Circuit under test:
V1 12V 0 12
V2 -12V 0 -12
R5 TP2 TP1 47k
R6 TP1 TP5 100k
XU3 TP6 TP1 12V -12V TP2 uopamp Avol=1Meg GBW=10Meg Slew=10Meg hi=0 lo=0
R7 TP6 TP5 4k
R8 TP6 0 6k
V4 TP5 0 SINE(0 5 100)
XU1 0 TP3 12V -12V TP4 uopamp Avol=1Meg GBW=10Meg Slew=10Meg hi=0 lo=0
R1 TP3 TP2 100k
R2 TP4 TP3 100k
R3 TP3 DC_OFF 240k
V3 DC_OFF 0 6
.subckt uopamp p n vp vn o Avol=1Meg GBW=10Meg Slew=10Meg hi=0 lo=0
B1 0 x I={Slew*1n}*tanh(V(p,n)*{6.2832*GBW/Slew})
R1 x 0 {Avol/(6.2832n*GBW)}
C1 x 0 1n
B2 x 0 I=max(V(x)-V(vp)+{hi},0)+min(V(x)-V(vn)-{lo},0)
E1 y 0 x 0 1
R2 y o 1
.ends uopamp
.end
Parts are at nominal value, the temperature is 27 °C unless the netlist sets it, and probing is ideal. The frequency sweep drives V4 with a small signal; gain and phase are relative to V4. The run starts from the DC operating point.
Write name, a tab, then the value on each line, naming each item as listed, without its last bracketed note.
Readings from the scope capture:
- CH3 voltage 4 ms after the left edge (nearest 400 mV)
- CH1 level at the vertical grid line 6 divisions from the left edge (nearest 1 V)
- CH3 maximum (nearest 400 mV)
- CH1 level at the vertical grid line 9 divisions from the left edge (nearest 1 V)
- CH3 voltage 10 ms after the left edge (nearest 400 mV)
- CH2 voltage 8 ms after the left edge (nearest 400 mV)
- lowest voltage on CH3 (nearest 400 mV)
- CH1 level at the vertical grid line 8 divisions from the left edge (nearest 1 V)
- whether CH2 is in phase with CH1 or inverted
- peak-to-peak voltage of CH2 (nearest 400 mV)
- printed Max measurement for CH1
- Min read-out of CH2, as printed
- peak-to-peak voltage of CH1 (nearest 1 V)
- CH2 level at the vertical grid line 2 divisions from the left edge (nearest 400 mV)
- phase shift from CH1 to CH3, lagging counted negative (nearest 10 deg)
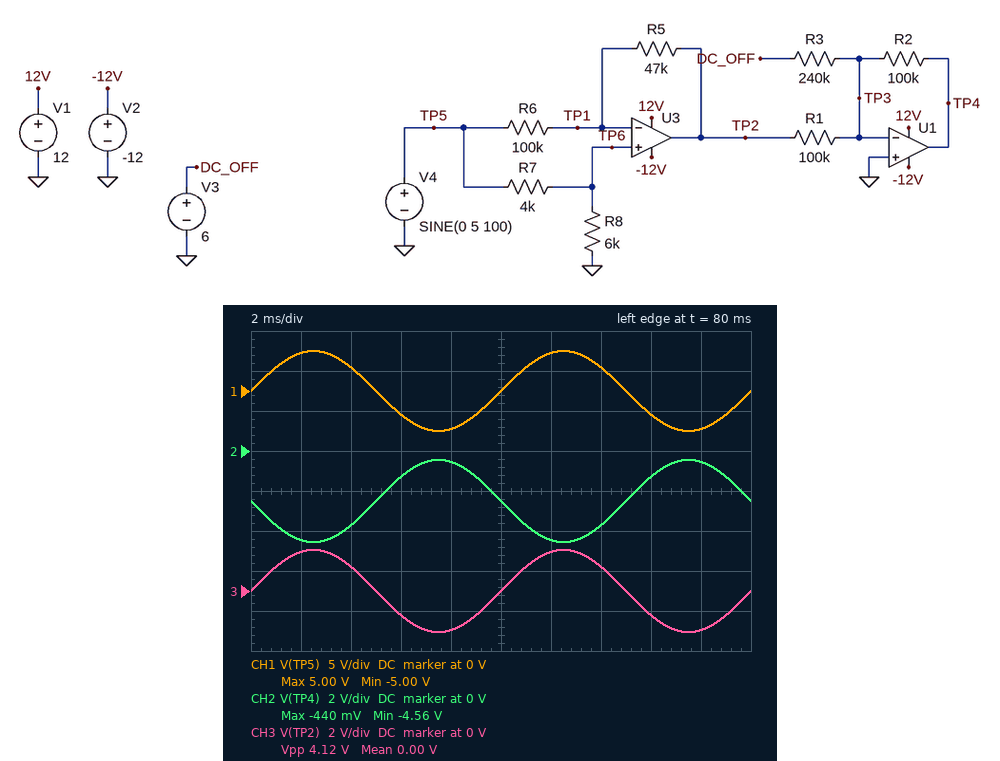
CH3 voltage 4 ms after the left edge	1.2 V
CH1 level at the vertical grid line 6 divisions from the left edge	5 V
CH3 maximum	2.0 V
CH1 level at the vertical grid line 9 divisions from the left edge	-5 V
CH3 voltage 10 ms after the left edge	0 V
CH2 voltage 8 ms after the left edge	-400 mV
lowest voltage on CH3	-2.0 V
CH1 level at the vertical grid line 8 divisions from the left edge	-3 V
whether CH2 is in phase with CH1 or inverted	inverted
peak-to-peak voltage of CH2	4.0 V
printed Max measurement for CH1	5.00 V
Min read-out of CH2, as printed	-4.56 V
peak-to-peak voltage of CH1	10 V
CH2 level at the vertical grid line 2 divisions from the left edge	-3.6 V
phase shift from CH1 to CH3, lagging counted negative	0 deg
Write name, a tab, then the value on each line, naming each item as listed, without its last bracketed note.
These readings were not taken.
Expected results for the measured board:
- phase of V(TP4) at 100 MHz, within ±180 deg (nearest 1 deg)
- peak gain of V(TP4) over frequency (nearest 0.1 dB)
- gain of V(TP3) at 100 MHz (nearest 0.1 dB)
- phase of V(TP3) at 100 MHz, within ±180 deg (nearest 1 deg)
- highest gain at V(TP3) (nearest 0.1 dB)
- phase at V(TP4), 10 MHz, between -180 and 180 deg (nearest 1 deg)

phase of V(TP4) at 100 MHz, within ±180 deg	6 deg
peak gain of V(TP4) over frequency	-7.7 dB
gain of V(TP3) at 100 MHz	-38.7 dB
phase of V(TP3) at 100 MHz, within ±180 deg	-84 deg
highest gain at V(TP3)	-19.5 dB
phase at V(TP4), 10 MHz, between -180 and 180 deg	57 deg
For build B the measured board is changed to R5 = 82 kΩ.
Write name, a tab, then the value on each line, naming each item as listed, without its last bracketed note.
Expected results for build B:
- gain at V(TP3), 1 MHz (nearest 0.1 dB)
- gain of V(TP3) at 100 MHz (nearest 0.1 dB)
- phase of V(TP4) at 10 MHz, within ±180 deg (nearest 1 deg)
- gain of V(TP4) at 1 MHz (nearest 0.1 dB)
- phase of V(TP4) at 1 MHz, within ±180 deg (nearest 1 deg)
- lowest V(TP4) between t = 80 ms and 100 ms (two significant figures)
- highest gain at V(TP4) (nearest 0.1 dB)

gain at V(TP3), 1 MHz	-31.7 dB
gain of V(TP3) at 100 MHz	-44.2 dB
phase of V(TP4) at 10 MHz, within ±180 deg	51 deg
gain of V(TP4) at 1 MHz	-11.7 dB
phase of V(TP4) at 1 MHz, within ±180 deg	156 deg
lowest V(TP4) between t = 80 ms and 100 ms	-3.9 V
highest gain at V(TP4)	-11.3 dB
